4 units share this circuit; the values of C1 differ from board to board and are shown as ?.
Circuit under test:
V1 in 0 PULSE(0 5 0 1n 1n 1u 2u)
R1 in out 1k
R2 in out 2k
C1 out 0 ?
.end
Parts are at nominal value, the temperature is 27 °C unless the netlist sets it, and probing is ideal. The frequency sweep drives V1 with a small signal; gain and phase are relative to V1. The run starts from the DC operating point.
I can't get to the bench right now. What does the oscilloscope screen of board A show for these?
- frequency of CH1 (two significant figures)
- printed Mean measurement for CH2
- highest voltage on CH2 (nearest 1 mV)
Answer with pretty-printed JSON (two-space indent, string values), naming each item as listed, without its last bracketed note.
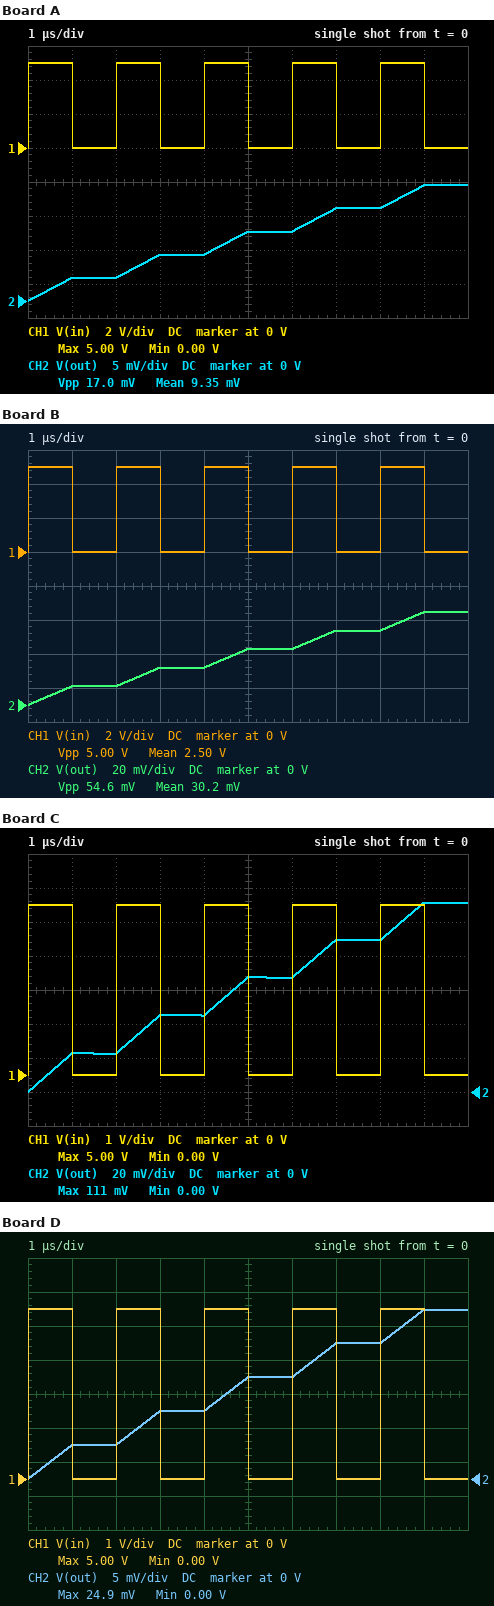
{
  "frequency of CH1": "500 kHz",
  "printed Mean measurement for CH2": "9.35 mV",
  "highest voltage on CH2": "17 mV"
}
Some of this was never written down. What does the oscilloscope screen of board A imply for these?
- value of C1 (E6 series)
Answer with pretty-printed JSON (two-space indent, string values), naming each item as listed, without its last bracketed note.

{
  "value of C1": "2.2 µF"
}
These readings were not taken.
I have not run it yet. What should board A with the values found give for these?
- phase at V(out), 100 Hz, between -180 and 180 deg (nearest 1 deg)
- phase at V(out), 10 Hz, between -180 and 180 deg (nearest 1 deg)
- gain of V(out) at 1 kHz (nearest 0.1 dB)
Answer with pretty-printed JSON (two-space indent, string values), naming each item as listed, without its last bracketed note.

{
  "phase at V(out), 100 Hz, between -180 and 180 deg": "-43 deg",
  "phase at V(out), 10 Hz, between -180 and 180 deg": "-5 deg",
  "gain of V(out) at 1 kHz": "-19.3 dB"
}
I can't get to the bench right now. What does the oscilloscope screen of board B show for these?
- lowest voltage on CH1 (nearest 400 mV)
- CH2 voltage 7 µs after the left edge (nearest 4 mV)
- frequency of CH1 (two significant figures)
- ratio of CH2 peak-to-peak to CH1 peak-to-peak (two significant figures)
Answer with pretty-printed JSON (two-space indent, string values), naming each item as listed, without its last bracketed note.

{
  "lowest voltage on CH1": "0 V",
  "CH2 voltage 7 µs after the left edge": "44 mV",
  "frequency of CH1": "500 kHz",
  "ratio of CH2 peak-to-peak to CH1 peak-to-peak": "0.011"
}
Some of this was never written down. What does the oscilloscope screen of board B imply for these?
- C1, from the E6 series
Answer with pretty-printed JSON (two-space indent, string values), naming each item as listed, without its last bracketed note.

{
  "C1, from the E6 series": "680 nF"
}
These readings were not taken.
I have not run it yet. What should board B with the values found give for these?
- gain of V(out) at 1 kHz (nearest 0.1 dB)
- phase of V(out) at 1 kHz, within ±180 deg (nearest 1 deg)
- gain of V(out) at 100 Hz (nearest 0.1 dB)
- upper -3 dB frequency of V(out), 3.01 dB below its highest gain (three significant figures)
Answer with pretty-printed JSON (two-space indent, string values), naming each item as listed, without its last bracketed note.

{
  "gain of V(out) at 1 kHz": "-9.6 dB",
  "phase of V(out) at 1 kHz, within ±180 deg": "-71 deg",
  "gain of V(out) at 100 Hz": "-0.3 dB",
  "upper -3 dB frequency of V(out), 3.01 dB below its highest gain": "351 Hz"
}
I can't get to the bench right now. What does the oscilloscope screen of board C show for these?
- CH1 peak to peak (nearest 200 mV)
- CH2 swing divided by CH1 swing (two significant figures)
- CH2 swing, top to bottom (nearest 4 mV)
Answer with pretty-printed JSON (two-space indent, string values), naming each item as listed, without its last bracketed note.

{
  "CH1 peak to peak": "5.0 V",
  "CH2 swing divided by CH1 swing": "0.022",
  "CH2 swing, top to bottom": "112 mV"
}
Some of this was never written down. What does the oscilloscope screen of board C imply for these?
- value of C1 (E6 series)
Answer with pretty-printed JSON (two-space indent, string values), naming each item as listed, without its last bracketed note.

{
  "value of C1": "330 nF"
}
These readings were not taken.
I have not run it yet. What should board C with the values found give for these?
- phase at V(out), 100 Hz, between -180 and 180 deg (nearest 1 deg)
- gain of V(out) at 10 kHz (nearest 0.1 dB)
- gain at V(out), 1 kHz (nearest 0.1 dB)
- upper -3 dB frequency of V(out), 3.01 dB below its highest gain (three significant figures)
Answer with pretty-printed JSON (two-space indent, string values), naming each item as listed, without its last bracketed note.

{
  "phase at V(out), 100 Hz, between -180 and 180 deg": "-8 deg",
  "gain of V(out) at 10 kHz": "-22.8 dB",
  "gain at V(out), 1 kHz": "-4.6 dB",
  "upper -3 dB frequency of V(out), 3.01 dB below its highest gain": "723 Hz"
}
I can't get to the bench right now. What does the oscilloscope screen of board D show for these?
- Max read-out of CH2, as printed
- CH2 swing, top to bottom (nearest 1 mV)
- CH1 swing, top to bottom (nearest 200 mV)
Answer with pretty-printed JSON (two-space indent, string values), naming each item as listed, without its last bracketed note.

{
  "Max read-out of CH2, as printed": "24.9 mV",
  "CH2 swing, top to bottom": "25 mV",
  "CH1 swing, top to bottom": "5.0 V"
}
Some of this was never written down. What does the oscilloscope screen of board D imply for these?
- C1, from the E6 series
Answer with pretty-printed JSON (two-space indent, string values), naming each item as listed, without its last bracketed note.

{
  "C1, from the E6 series": "1.5 µF"
}
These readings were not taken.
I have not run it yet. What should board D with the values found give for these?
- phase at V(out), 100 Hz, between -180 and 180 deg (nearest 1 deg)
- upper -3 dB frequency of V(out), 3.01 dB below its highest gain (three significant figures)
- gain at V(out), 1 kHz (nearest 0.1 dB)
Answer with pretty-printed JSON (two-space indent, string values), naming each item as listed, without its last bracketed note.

{
  "phase at V(out), 100 Hz, between -180 and 180 deg": "-32 deg",
  "upper -3 dB frequency of V(out), 3.01 dB below its highest gain": "159 Hz",
  "gain at V(out), 1 kHz": "-16.1 dB"
}
